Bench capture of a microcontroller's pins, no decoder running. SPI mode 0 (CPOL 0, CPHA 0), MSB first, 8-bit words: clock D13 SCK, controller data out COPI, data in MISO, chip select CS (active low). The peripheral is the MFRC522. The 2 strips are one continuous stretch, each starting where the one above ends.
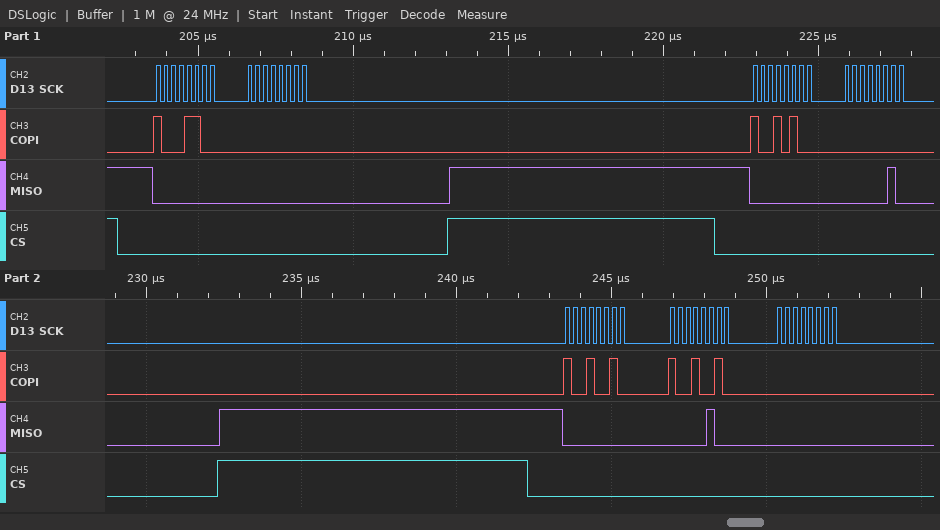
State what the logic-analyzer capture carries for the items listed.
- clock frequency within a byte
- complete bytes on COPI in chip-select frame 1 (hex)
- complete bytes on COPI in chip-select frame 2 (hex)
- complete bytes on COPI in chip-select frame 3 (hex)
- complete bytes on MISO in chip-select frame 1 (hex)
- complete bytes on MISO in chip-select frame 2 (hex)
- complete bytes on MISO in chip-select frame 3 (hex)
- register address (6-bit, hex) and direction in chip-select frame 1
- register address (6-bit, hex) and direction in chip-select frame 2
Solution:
4 MHz
8C 00
94 00
92 92 00
00 00
00 02
00 04 00
0x06 read
0x0A read
